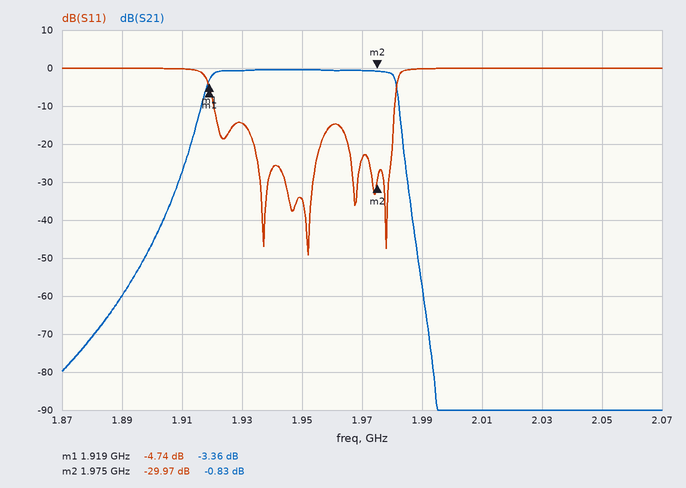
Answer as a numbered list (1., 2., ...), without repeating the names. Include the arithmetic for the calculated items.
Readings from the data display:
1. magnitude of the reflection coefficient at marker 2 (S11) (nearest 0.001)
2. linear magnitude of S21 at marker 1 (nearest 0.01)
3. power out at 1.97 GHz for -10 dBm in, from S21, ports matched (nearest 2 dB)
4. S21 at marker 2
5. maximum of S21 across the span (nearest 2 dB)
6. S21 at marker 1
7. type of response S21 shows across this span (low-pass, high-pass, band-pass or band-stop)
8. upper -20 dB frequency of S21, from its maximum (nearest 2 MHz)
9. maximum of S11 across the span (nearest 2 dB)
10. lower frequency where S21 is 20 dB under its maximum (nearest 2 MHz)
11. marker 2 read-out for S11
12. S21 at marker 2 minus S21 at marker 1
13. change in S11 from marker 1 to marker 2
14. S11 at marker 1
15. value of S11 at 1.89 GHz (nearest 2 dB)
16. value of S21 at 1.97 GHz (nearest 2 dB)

1. 10^(-29.97/20) ≈ 0.032
2. 10^(-3.36/20) ≈ 0.68
3. -10 dBm + (0 dB) = -10 dBm
4. -0.83 dB
5. 0 dB
6. -3.36 dB
7. band-pass
8. 1.984 GHz
9. 0 dB
10. 1.912 GHz
11. -29.97 dB
12. -0.83 − (-3.36) = 2.53 dB
13. -29.97 − (-4.74) = -25.23 dB
14. -4.74 dB
15. 0 dB
16. 0 dB
